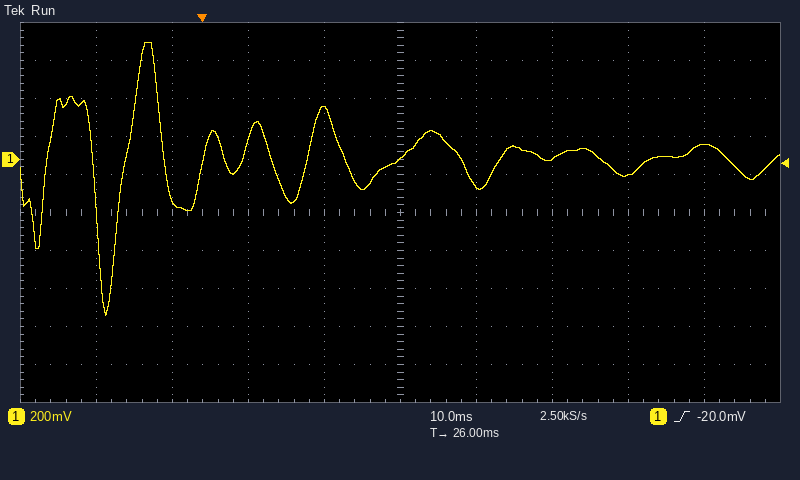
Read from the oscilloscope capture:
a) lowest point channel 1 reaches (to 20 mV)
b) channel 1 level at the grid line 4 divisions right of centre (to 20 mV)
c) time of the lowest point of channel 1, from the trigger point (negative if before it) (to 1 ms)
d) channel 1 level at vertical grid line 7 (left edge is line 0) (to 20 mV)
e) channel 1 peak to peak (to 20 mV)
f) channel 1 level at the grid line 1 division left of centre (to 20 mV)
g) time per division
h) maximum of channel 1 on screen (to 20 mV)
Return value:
-820 mV
80 mV
-13 ms
0 mV
1.44 V
260 mV
10 ms
620 mV
